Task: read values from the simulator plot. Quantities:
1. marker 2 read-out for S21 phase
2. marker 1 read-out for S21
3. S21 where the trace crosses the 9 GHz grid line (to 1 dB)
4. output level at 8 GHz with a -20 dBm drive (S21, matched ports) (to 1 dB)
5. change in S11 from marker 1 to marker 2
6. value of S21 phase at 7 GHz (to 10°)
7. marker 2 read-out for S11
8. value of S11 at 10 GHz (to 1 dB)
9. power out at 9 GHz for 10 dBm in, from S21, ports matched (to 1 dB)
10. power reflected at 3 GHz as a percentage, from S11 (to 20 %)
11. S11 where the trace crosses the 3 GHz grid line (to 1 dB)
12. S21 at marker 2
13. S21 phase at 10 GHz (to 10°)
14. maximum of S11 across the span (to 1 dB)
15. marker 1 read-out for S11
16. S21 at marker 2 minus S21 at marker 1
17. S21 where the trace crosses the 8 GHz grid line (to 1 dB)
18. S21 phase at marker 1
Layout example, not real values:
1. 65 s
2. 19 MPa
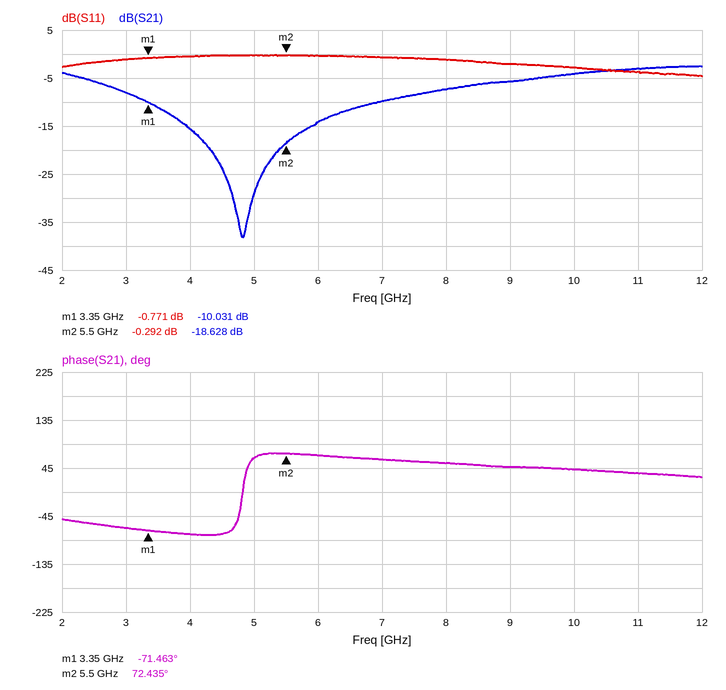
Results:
1. 72.435°
2. -10.031 dB
3. -6 dB
4. -27 dBm
5. 0.479 dB
6. 60°
7. -0.292 dB
8. -3 dB
9. 4 dBm
10. 80 %
11. -1 dB
12. -18.628 dB
13. 40°
14. 0 dB
15. -0.771 dB
16. -8.597 dB
17. -7 dB
18. -71.463°
